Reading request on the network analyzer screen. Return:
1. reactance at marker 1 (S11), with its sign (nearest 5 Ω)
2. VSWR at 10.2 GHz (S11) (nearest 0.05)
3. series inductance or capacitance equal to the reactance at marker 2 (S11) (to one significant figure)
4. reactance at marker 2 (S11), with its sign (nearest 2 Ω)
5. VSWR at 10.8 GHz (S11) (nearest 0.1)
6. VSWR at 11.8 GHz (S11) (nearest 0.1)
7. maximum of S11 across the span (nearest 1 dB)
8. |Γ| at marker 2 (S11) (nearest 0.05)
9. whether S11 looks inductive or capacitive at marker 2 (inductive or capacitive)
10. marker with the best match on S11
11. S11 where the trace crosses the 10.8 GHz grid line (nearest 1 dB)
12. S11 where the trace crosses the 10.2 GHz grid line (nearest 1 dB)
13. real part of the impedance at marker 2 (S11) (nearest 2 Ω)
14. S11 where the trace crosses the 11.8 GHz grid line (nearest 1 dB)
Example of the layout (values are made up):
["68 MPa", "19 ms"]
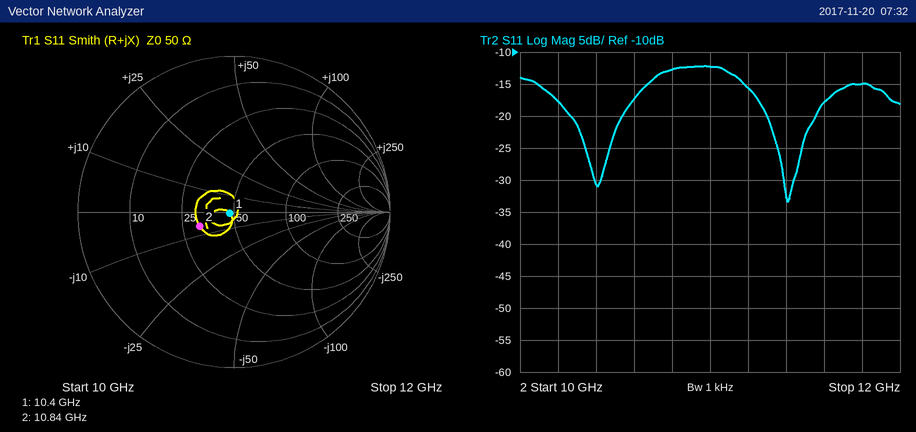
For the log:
["0 Ω", "1.30", "2 pF", "-6 Ω", "1.6", "1.4", "-12 dB", "0.25", "capacitive", "marker 1", "-13 dB", "-18 dB", "32 Ω", "-15 dB"]
